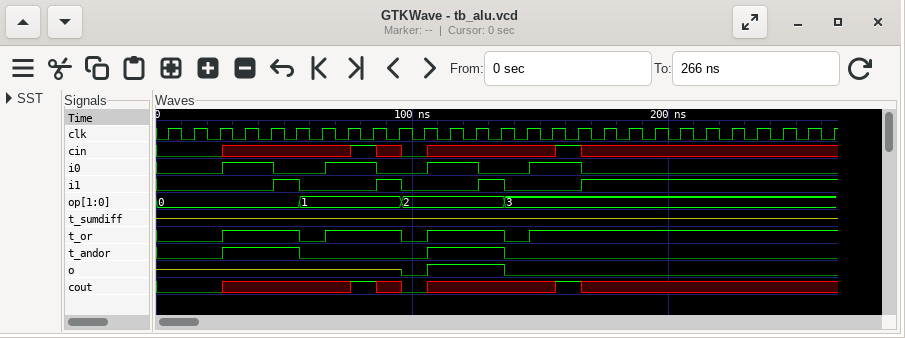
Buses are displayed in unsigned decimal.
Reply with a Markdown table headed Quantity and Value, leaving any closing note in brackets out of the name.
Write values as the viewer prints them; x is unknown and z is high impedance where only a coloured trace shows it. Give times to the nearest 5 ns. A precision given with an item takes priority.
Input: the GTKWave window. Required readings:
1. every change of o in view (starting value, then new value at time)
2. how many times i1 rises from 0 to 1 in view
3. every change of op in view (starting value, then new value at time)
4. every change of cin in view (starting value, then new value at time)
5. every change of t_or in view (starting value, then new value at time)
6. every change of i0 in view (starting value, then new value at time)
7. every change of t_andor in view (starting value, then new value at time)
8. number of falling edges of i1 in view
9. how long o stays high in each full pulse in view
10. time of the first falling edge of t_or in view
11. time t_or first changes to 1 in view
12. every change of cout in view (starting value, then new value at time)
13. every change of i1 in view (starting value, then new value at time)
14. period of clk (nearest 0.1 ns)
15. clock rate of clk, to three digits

| Quantity | Value |
|---|---|
| every change of o in view | z, 0 at 95 ns, 1 at 105 ns, 0 at 135 ns |
| how many times i1 rises from 0 to 1 in view | 4 |
| every change of op in view | 0, 1 at 55 ns, 2 at 95 ns, 3 at 135 ns |
| every change of cin in view | 0, x at 25 ns, 1 at 75 ns, x at 85 ns, 0 at 95 ns, x at 105 ns, 1 at 155 ns, x at 165 ns |
| every change of t_or in view | 0, 1 at 25 ns, 0 at 55 ns, 1 at 65 ns, 0 at 95 ns, 1 at 105 ns, 0 at 135 ns, 1 at 145 ns |
| every change of i0 in view | 0, 1 at 25 ns, 0 at 45 ns, 1 at 65 ns, 0 at 85 ns, 1 at 105 ns, 0 at 125 ns, 1 at 145 ns, 0 at 165 ns |
| every change of t_andor in view | 0, 1 at 25 ns, 0 at 55 ns, 1 at 105 ns, 0 at 135 ns |
| number of falling edges of i1 in view | 3 |
| how long o stays high in each full pulse in view | 30 ns |
| time of the first falling edge of t_or in view | 55 ns |
| time t_or first changes to 1 in view | 25 ns |
| every change of cout in view | 0, x at 25 ns, 1 at 75 ns, x at 85 ns, 0 at 95 ns, x at 105 ns, 1 at 155 ns, x at 165 ns |
| every change of i1 in view | 0, 1 at 45 ns, 0 at 55 ns, 1 at 85 ns, 0 at 95 ns, 1 at 125 ns, 0 at 135 ns, 1 at 165 ns |
| period of clk | 10 ns |
| clock rate of clk, to three digits | 100 MHz |
